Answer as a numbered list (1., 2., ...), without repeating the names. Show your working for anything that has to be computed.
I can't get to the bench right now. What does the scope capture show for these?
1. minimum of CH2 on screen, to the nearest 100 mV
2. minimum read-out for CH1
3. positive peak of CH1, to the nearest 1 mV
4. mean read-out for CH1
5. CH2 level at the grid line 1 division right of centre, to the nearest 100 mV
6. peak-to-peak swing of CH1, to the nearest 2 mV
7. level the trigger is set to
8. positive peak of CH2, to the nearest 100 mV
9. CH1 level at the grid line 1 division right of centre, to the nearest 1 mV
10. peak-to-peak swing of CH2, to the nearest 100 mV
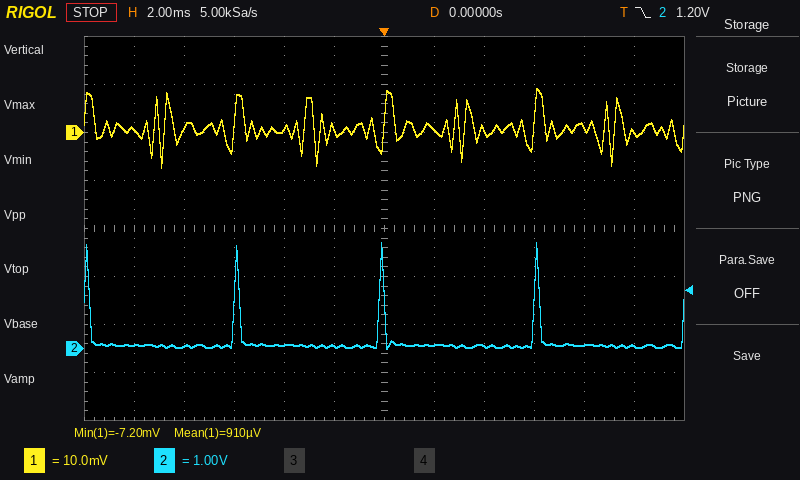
1. 0.0 V
2. -7.20 mV
3. 9 mV
4. 910 µV
5. 100 mV
6. 16 mV
7. 1.20 V
8. 2.2 V
9. 1 mV
10. 2.2 V − (0.0 V) = 2.2 V
